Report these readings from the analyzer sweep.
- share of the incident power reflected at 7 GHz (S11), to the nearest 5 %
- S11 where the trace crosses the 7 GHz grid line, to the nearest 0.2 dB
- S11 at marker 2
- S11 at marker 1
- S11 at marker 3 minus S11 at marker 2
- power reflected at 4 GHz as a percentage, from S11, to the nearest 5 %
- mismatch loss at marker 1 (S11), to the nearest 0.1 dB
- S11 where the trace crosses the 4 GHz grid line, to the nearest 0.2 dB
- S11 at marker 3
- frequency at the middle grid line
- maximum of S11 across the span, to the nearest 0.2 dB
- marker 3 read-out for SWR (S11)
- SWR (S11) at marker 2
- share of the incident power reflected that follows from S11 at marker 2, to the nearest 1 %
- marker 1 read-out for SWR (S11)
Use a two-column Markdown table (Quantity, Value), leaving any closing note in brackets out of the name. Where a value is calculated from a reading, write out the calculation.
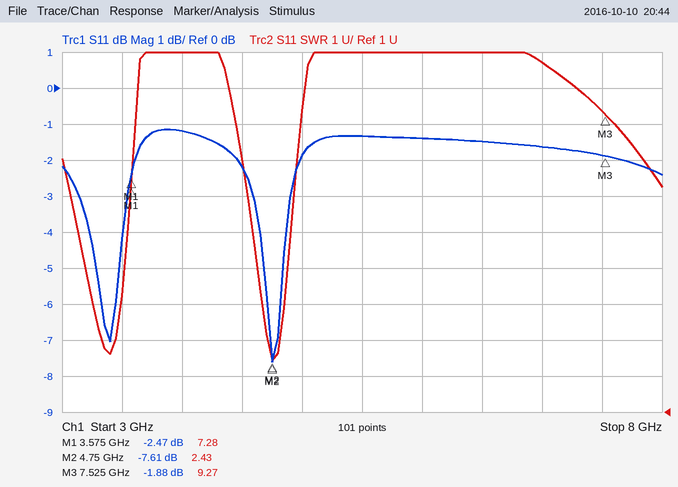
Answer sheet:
| Quantity | Value |
|---|---|
| share of the incident power reflected at 7 GHz (S11), to the nearest 5 % | 10^(-1.6/10) ≈ 69.2 %, so 70 % to the nearest 5 % |
| S11 where the trace crosses the 7 GHz grid line, to the nearest 0.2 dB | -1.6 dB |
| S11 at marker 2 | -7.61 dB |
| S11 at marker 1 | -2.47 dB |
| S11 at marker 3 minus S11 at marker 2 | -1.88 − (-7.61) = 5.73 dB |
| power reflected at 4 GHz as a percentage, from S11, to the nearest 5 % | 10^(-1.2/10) ≈ 75.9 %, so 75 % to the nearest 5 % |
| mismatch loss at marker 1 (S11), to the nearest 0.1 dB | −10 log10(1 − 10^(-2.47/10)) ≈ 3.6 dB |
| S11 where the trace crosses the 4 GHz grid line, to the nearest 0.2 dB | -1.2 dB |
| S11 at marker 3 | -1.88 dB |
| frequency at the middle grid line | 5.5 GHz |
| maximum of S11 across the span, to the nearest 0.2 dB | -1.2 dB |
| marker 3 read-out for SWR | 9.27 |
| SWR (S11) at marker 2 | 2.43 |
| share of the incident power reflected that follows from S11 at marker 2, to the nearest 1 % | 10^(-7.61/10) ≈ 17 % |
| marker 1 read-out for SWR | 7.28 |
